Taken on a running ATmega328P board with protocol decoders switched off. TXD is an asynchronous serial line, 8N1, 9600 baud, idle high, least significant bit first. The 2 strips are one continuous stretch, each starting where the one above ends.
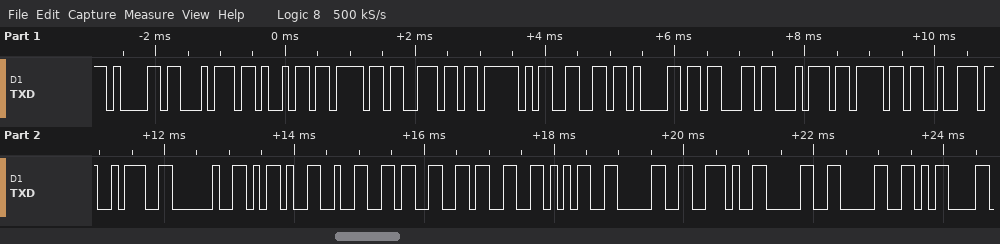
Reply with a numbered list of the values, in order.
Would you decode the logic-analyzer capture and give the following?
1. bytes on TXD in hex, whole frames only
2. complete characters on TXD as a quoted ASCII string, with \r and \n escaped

1. 0x61 0x74 0x69 0x6F 0x6E 0x5F 0x66 0x61 0x63 0x74 0x6F 0x72 0x3A 0x20 0x2D 0x32 0x33 0x33 0x35 0x30 0x2E 0x30 0x30 0x0D
2. "ation_factor: -23350.00\r"
